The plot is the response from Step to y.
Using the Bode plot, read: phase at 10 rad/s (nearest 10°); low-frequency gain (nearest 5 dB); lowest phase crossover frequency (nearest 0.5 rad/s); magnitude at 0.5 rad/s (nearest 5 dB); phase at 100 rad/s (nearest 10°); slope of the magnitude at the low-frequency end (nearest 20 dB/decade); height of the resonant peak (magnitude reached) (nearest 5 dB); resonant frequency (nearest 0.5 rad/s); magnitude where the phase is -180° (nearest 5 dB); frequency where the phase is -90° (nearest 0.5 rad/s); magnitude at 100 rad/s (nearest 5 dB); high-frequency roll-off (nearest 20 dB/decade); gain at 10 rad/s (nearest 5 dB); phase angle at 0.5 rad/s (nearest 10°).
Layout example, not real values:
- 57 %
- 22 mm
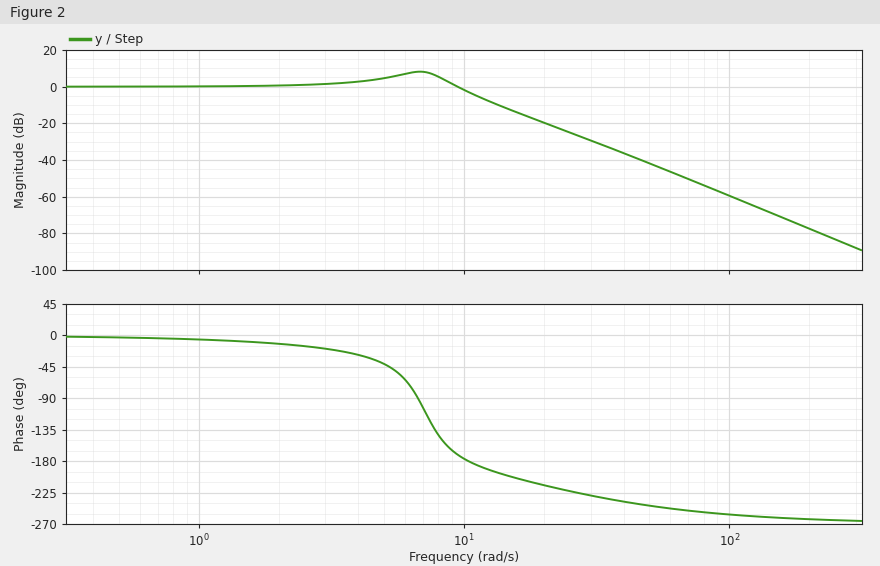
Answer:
- -180°
- 0 dB
- 10.5 rad/s
- 0 dB
- -260°
- 0 dB/decade
- 10 dB
- 7.0 rad/s
- -5 dB
- 6.5 rad/s
- -60 dB
- -60 dB/decade
- 0 dB
- 0°
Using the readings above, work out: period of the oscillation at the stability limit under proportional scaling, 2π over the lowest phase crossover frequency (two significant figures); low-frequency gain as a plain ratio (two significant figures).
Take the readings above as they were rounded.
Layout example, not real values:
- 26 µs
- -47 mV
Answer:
- 0.60 s
- 1.0
